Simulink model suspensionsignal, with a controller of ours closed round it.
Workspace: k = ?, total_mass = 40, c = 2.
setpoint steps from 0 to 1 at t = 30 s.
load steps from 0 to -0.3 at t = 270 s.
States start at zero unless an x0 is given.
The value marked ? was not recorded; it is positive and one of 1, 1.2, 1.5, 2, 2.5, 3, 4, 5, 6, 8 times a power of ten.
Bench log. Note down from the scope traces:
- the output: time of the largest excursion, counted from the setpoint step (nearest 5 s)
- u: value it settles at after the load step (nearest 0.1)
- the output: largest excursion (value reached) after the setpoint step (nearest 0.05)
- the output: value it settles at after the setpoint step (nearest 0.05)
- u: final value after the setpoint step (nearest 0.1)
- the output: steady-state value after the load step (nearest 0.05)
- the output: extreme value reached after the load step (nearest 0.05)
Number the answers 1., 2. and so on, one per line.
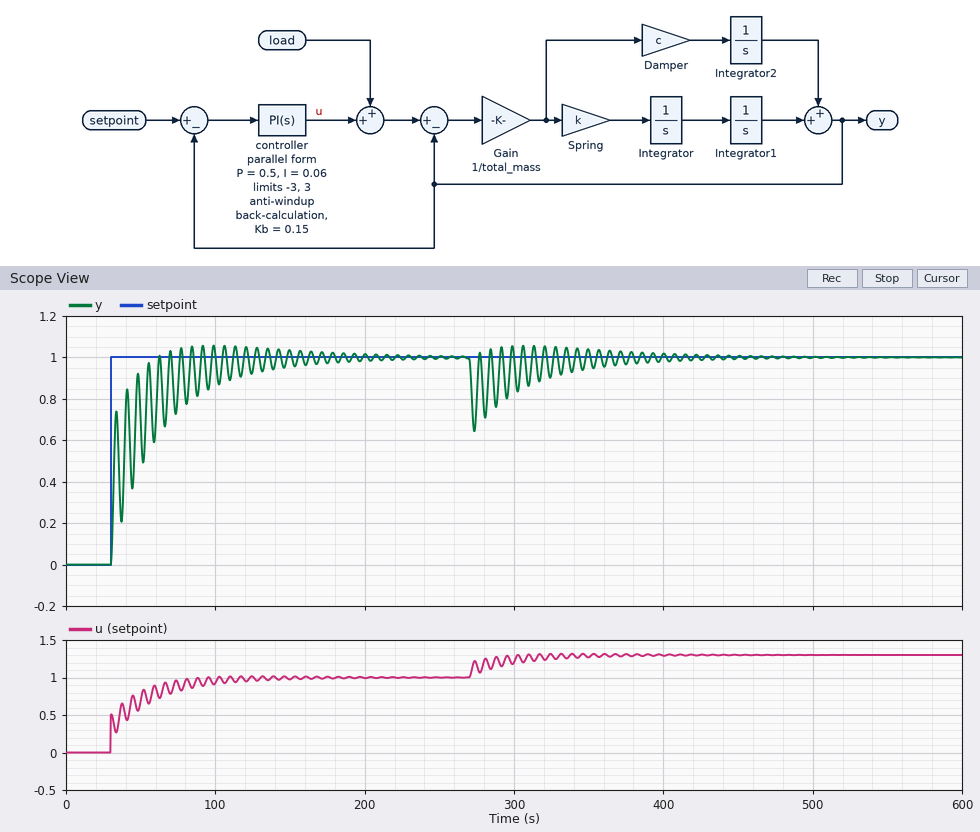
1. 70 s
2. 1.3
3. 1.05
4. 1.00
5. 1.0
6. 1.00
7. 0.65
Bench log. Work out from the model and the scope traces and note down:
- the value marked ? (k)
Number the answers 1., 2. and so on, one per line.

1. 20
